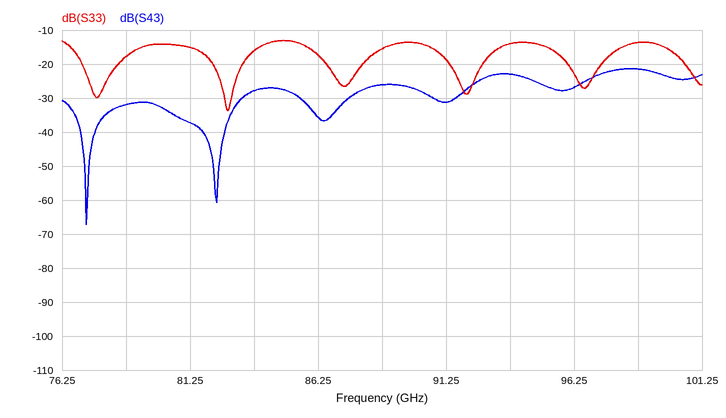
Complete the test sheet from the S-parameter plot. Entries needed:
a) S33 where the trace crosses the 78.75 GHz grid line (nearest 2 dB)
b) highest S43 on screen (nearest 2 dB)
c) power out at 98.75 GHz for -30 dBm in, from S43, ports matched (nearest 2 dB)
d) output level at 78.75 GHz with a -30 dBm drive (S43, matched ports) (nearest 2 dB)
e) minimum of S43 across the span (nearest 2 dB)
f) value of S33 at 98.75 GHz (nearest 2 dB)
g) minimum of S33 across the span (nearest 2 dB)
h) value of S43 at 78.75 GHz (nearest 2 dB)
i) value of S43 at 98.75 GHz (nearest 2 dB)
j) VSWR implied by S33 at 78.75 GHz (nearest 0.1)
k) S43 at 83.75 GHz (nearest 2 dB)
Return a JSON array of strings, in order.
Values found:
["-18 dB", "-22 dB", "-52 dBm", "-62 dBm", "-68 dB", "-14 dB", "-34 dB", "-32 dB", "-22 dB", "1.3", "-28 dB"]
